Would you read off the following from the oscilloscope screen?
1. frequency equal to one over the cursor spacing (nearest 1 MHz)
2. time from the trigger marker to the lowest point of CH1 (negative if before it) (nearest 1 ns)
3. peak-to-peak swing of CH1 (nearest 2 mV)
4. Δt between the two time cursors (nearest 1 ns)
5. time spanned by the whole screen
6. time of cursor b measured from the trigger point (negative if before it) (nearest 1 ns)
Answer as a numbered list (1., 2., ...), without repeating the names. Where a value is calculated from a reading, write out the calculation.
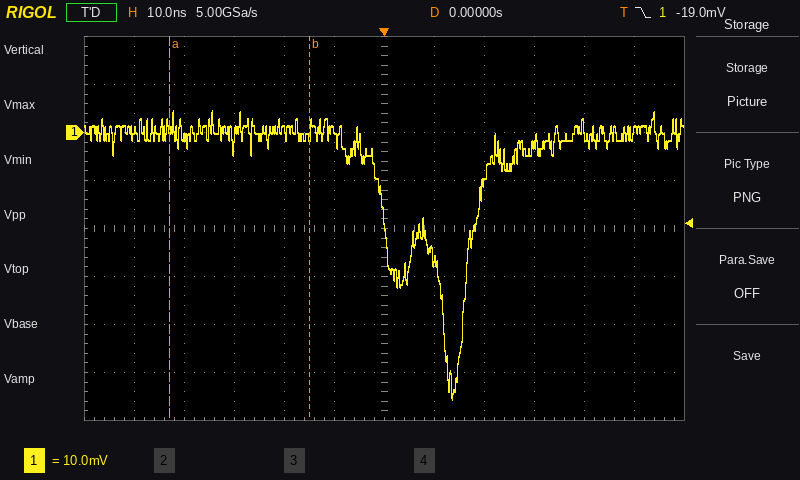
1. 1 / 28 ns ≈ 36 MHz
2. +14 ns
3. 60 mV
4. 28 ns
5. 120 ns
6. -15 ns
